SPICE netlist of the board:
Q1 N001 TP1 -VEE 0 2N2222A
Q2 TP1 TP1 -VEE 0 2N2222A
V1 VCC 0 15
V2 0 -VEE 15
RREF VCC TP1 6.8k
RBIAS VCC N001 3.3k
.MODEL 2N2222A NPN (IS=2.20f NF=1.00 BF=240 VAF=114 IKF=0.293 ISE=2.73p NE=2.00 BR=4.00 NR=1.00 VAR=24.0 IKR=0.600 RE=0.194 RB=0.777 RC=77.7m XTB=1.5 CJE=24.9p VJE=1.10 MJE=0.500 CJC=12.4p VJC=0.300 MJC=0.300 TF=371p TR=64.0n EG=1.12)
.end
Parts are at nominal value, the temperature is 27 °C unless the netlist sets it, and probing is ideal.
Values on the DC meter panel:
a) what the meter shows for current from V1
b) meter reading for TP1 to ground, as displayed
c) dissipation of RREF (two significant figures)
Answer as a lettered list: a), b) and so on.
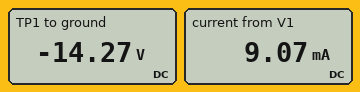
a) 9.07 mA
b) -14.27 V
c) 130 mW
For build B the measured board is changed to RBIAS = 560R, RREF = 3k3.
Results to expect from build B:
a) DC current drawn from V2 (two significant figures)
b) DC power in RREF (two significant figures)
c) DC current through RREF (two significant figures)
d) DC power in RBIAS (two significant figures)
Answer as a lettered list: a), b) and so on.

a) 19 mA
b) 260 mW
c) 8.9 mA
d) 62 mW
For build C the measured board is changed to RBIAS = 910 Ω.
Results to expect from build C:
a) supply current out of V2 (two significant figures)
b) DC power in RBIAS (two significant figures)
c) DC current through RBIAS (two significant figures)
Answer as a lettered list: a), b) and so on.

a) 9.5 mA
b) 24 mW
c) 5.2 mA
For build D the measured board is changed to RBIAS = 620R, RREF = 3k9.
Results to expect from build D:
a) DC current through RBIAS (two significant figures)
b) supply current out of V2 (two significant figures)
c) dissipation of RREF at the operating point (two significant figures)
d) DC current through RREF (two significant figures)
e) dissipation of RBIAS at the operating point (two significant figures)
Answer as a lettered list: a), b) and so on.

a) 8.9 mA
b) 16 mA
c) 220 mW
d) 7.5 mA
e) 49 mW
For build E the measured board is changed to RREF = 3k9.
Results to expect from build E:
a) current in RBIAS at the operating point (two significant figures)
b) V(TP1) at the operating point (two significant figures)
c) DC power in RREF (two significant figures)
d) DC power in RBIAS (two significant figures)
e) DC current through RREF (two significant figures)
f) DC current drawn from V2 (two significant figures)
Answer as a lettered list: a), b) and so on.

a) 7.7 mA
b) -14 V
c) 220 mW
d) 190 mW
e) 7.5 mA
f) 15 mA
